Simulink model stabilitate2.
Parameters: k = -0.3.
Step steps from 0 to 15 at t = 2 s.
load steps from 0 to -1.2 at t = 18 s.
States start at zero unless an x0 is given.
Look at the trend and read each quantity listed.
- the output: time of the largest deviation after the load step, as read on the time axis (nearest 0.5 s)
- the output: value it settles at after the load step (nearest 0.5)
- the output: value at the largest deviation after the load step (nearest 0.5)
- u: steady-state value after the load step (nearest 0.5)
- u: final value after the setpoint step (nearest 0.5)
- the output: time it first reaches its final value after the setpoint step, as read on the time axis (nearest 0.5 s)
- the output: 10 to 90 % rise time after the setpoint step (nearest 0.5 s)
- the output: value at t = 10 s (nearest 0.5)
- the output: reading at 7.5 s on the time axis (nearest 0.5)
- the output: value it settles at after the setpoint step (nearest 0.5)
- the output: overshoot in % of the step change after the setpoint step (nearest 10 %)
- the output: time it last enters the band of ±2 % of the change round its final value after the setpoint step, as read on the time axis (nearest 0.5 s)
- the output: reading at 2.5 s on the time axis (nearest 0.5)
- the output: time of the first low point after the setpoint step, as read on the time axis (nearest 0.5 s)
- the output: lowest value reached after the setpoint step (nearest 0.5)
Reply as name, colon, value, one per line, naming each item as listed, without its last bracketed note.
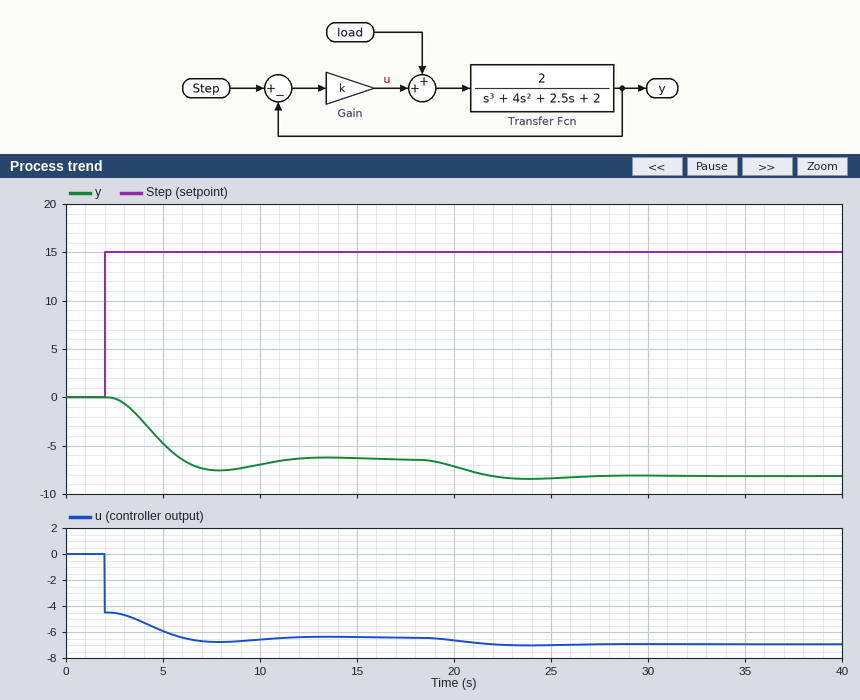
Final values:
the output: time of the largest deviation after the load step, as read on the time axis: 24.0 s
the output: value it settles at after the load step: -8.0
the output: value at the largest deviation after the load step: -8.5
u: steady-state value after the load step: -7.0
u: final value after the setpoint step: -6.5
the output: time it first reaches its final value after the setpoint step, as read on the time axis: 6.0 s
the output: 10 to 90 % rise time after the setpoint step: 2.5 s
the output: value at t = 10 s: -7.0
the output: reading at 7.5 s on the time axis: -7.5
the output: value it settles at after the setpoint step: -6.5
the output: overshoot in % of the step change after the setpoint step: 20 %
the output: time it last enters the band of ±2 % of the change round its final value after the setpoint step, as read on the time axis: 15.0 s
the output: reading at 2.5 s on the time axis: 0.0
the output: time of the first low point after the setpoint step, as read on the time axis: 8.0 s
the output: lowest value reached after the setpoint step: -7.5
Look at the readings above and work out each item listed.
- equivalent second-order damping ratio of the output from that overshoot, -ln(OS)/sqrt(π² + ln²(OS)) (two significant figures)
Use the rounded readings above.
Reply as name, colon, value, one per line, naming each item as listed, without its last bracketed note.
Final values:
equivalent second-order damping ratio of the output from that overshoot, -ln(OS)/sqrt(π² + ln²(OS)): 0.46
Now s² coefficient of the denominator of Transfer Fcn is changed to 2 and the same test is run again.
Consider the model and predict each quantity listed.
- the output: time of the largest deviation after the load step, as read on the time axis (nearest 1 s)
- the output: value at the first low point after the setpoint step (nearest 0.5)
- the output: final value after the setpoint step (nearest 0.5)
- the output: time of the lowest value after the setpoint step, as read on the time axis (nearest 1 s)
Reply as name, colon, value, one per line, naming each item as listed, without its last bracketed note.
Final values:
the output: time of the largest deviation after the load step, as read on the time axis: 22 s
the output: value at the first low point after the setpoint step: -7.0
the output: final value after the setpoint step: -6.5
the output: time of the lowest value after the setpoint step, as read on the time axis: 6 s
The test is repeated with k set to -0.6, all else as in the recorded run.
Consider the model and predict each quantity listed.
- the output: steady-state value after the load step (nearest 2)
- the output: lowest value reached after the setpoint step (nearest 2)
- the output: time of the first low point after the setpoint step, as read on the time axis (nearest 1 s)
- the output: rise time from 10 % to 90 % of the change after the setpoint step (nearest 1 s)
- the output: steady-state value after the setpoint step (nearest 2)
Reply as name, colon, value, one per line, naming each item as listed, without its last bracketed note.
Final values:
the output: steady-state value after the load step: -26
the output: lowest value reached after the setpoint step: -24
the output: time of the first low point after the setpoint step, as read on the time axis: 11 s
the output: rise time from 10 % to 90 % of the change after the setpoint step: 4 s
the output: steady-state value after the setpoint step: -22
